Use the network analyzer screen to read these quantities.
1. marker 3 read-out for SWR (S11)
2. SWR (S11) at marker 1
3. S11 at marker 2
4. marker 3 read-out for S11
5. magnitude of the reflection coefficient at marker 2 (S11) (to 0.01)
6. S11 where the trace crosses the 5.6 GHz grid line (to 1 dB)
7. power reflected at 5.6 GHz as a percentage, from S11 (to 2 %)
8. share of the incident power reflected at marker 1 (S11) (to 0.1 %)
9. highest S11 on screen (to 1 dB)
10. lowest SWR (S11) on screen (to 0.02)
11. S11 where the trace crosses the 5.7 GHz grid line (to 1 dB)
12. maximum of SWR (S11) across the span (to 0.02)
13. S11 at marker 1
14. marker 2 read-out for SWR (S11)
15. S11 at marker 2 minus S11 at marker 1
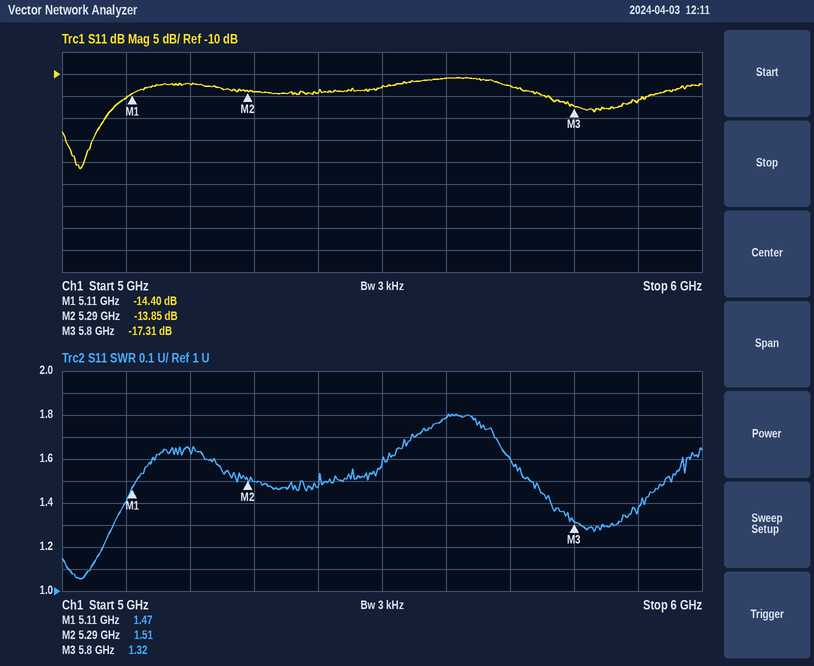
1.32
1.47
-13.85 dB
-17.31 dB
0.20
-11 dB
8 %
3.6 %
-11 dB
1.06
-13 dB
1.80
-14.40 dB
1.51
0.55 dB
